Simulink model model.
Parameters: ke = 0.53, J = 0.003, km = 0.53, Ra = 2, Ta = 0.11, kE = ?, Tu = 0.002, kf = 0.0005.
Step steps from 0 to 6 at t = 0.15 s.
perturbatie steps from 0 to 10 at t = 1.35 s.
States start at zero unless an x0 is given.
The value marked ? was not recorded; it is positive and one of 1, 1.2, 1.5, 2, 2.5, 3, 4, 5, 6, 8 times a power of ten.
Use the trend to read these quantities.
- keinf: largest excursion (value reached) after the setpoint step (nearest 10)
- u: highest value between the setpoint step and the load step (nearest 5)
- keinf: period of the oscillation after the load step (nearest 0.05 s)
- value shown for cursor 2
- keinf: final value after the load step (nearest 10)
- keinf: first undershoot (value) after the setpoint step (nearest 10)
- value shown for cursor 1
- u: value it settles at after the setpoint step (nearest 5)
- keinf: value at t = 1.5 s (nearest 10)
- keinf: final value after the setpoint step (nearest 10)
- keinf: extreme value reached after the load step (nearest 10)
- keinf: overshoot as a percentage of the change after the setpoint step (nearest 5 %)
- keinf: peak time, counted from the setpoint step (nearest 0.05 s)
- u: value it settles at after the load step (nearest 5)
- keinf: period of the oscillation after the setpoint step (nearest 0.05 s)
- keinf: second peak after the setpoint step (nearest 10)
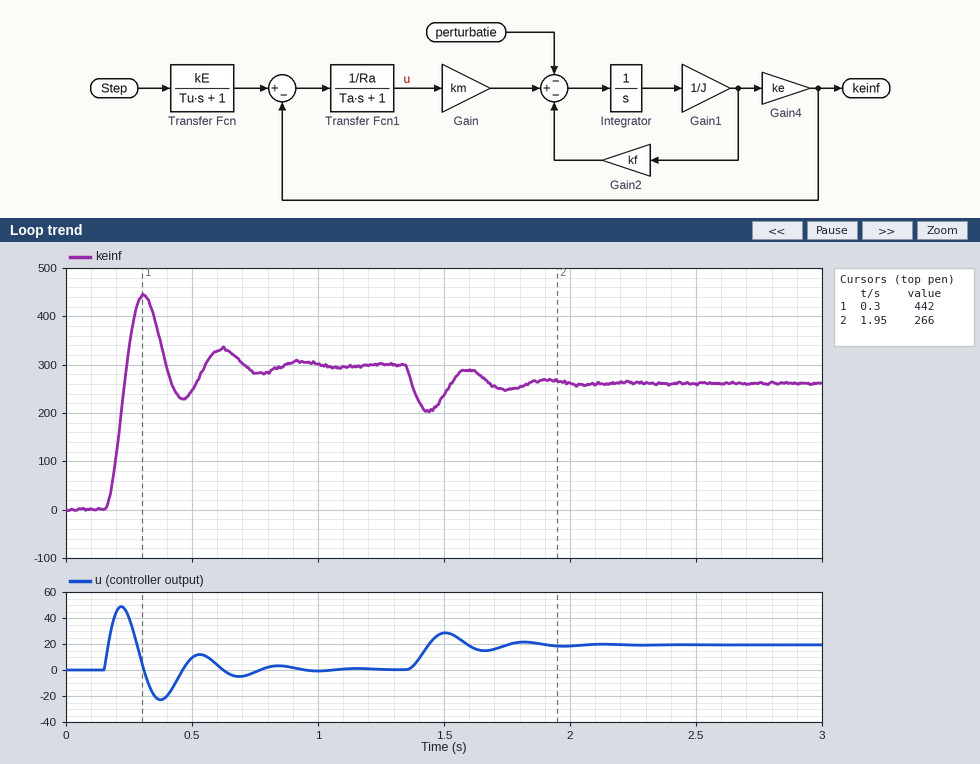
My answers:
440
50
0.30 s
266
260
230
442
0
240
300
200
50 %
0.15 s
20
0.30 s
330
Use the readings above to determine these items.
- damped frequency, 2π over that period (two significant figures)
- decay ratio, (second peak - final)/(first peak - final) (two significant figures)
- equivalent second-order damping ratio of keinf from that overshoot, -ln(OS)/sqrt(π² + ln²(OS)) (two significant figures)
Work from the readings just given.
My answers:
21 rad/s
0.21
0.22
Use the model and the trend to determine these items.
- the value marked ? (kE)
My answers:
50
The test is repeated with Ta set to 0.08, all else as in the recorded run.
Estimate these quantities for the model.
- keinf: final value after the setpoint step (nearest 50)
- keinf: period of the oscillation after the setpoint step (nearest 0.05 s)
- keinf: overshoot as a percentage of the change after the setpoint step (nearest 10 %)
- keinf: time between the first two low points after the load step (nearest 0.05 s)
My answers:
300
0.25 s
40 %
0.25 s
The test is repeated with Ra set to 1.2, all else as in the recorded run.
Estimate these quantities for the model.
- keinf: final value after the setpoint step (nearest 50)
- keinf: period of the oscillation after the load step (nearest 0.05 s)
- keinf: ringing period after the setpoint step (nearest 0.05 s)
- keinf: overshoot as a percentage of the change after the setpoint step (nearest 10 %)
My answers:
300
0.25 s
0.25 s
60 %
